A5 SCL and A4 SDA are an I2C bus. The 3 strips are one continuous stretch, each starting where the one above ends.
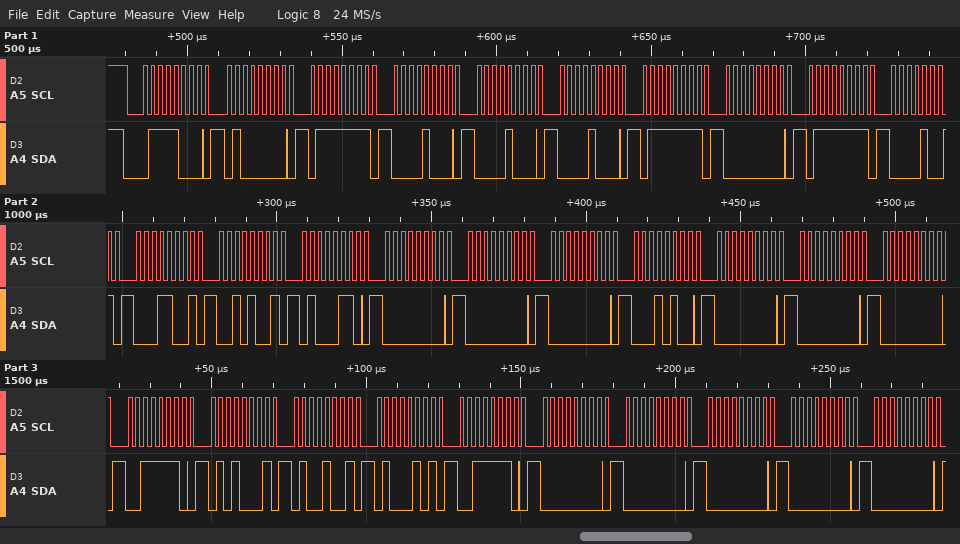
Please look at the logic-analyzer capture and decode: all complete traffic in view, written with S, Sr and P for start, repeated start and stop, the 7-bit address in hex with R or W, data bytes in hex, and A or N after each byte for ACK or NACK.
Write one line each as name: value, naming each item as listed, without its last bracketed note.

all complete traffic in view, written with S, Sr and P for start, repeated start and stop, the 7-bit address in hex with R or W, data bytes in hex, and A or N after each byte for ACK or NACK: S 3CW A 40 A 7F A 08 A 08 A 08 A 7F A 00 A 7F A 09 A 19 A 29 A 46 A 00 A 00 A 00 A 14 A 00 A 00 A 00 A 3E A 51 A 49 A 45 A 3E A 00 A 00 A 00 A 00 A 00 A
